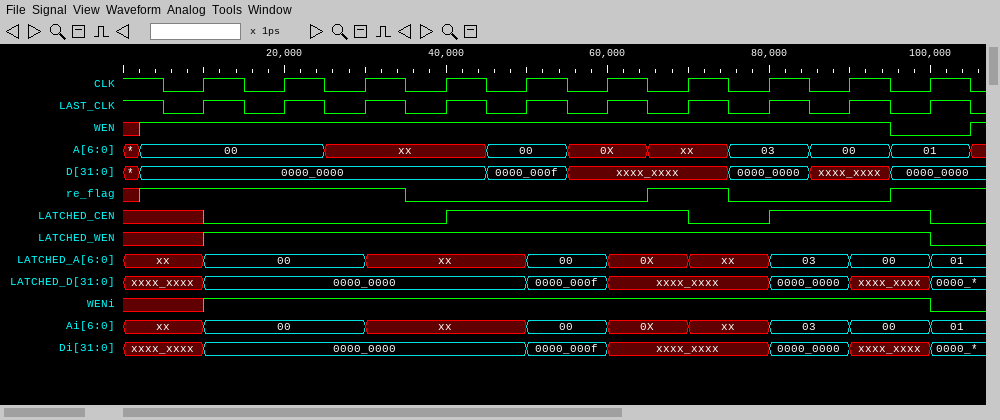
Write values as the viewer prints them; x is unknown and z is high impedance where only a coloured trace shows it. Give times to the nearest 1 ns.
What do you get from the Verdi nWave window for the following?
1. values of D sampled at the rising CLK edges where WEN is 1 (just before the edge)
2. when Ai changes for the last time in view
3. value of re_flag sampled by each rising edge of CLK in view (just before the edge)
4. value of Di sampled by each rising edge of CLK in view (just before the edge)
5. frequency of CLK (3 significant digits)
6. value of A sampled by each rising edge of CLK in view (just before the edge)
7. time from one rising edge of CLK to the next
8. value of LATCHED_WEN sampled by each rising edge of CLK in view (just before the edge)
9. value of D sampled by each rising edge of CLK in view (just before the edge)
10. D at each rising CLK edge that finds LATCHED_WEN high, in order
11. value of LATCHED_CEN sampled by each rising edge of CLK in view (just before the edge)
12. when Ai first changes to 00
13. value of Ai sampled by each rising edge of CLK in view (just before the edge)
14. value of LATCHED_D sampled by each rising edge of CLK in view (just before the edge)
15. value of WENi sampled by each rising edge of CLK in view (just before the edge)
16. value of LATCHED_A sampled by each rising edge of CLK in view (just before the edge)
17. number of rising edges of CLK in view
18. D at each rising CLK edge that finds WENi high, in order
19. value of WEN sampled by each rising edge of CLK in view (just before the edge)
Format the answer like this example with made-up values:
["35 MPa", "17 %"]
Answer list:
["0000_0000, 0000_0000, 0000_0000, 0000_0000, 0000_000f, xxxx_xxxx, xxxx_xxxx, 0000_0000, xxxx_xxxx", "100 ns", "1 1 1 0 0 0 1 0 0 1", "xxxx_xxxx, 0000_0000, 0000_0000, 0000_0000, 0000_0000, 0000_000f, xxxx_xxxx, xxxx_xxxx, 0000_0000, xxxx_xxxx", "100 MHz", "00, 00, xx, xx, 00, 0X, xx, 03, 00, 01", "10 ns", "x 1 1 1 1 1 1 1 1 1", "0000_0000, 0000_0000, 0000_0000, 0000_0000, 0000_000f, xxxx_xxxx, xxxx_xxxx, 0000_0000, xxxx_xxxx, 0000_0000", "0000_0000, 0000_0000, 0000_0000, 0000_000f, xxxx_xxxx, xxxx_xxxx, 0000_0000, xxxx_xxxx, 0000_0000", "x 0 0 0 1 1 1 0 1 1", "10 ns", "xx, 00, 00, xx, xx, 00, 0X, xx, 03, 00", "xxxx_xxxx, 0000_0000, 0000_0000, 0000_0000, 0000_0000, 0000_000f, xxxx_xxxx, xxxx_xxxx, 0000_0000, xxxx_xxxx", "x 1 1 1 1 1 1 1 1 1", "xx, 00, 00, xx, xx, 00, 0X, xx, 03, 00", "10", "0000_0000, 0000_0000, 0000_0000, 0000_000f, xxxx_xxxx, xxxx_xxxx, 0000_0000, xxxx_xxxx, 0000_0000", "1 1 1 1 1 1 1 1 1 0"]
